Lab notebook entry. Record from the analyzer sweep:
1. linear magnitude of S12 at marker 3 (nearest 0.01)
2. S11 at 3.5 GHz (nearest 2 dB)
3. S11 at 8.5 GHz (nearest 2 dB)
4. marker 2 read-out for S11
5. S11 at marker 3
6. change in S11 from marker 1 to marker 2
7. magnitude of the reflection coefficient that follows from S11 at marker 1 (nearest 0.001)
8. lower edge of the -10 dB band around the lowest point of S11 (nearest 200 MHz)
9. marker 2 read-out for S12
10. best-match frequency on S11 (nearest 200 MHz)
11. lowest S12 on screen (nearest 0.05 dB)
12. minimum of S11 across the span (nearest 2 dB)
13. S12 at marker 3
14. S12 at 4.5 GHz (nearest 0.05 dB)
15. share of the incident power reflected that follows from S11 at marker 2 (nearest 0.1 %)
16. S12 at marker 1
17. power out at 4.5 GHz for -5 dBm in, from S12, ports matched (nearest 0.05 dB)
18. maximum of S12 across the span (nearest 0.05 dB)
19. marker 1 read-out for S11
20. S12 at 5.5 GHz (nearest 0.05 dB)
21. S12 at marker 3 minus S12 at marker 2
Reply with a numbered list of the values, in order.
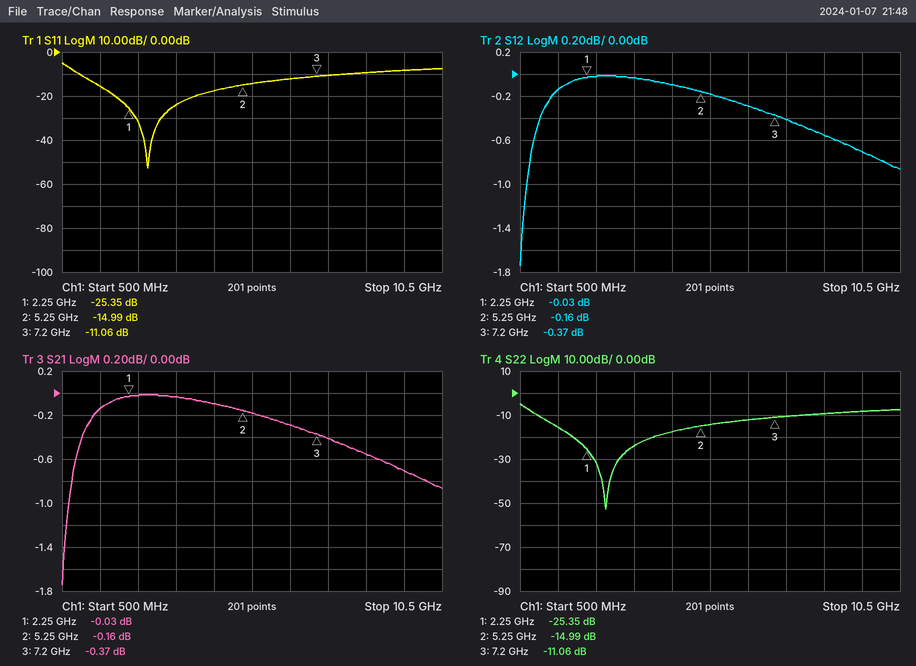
1. 0.96
2. -24 dB
3. -10 dB
4. -14.99 dB
5. -11.06 dB
6. 10.36 dB
7. 0.054
8. 1.0 GHz
9. -0.16 dB
10. 2.8 GHz
11. -1.75 dB
12. -52 dB
13. -0.37 dB
14. -0.10 dB
15. 3.2 %
16. -0.03 dB
17. -5.10 dBm
18. 0.00 dB
19. -25.35 dB
20. -0.20 dB
21. -0.21 dB
